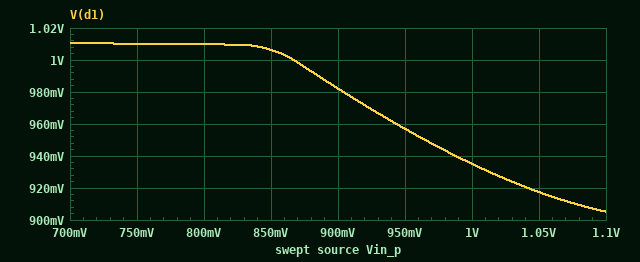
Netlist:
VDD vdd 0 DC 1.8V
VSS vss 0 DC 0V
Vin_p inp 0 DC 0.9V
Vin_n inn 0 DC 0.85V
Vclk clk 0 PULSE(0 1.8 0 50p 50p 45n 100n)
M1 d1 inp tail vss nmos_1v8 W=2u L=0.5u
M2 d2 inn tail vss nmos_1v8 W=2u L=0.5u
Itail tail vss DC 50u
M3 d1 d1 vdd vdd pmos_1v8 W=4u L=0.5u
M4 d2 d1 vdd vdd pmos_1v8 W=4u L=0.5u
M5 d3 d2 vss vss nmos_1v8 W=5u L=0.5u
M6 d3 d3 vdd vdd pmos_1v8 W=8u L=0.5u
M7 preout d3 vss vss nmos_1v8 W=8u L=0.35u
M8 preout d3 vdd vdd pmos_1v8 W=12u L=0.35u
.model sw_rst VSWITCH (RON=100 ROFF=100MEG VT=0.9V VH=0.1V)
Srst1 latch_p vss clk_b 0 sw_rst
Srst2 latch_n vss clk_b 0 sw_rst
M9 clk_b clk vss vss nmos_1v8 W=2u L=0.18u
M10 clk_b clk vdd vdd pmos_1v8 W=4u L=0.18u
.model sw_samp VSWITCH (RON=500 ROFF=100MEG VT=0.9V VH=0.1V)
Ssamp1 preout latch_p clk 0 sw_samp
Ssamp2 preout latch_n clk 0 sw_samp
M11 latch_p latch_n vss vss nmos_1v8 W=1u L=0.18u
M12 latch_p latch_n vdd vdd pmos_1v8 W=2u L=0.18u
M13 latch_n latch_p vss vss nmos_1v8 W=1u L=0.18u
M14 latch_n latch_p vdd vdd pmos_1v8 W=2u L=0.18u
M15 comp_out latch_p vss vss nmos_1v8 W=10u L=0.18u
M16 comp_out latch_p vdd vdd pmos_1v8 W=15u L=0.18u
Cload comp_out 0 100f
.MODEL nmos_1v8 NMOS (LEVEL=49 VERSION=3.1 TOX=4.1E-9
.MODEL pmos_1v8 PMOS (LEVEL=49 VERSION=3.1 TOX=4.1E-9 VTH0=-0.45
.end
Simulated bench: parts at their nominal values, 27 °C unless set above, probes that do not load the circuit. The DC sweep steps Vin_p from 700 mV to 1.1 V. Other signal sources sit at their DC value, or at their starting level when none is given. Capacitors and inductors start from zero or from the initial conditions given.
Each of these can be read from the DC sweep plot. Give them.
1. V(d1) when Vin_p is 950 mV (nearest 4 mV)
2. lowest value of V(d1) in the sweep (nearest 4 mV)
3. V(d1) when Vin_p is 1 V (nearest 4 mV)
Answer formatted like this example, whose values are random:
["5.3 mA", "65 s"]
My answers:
["956 mV", "904 mV", "936 mV"]
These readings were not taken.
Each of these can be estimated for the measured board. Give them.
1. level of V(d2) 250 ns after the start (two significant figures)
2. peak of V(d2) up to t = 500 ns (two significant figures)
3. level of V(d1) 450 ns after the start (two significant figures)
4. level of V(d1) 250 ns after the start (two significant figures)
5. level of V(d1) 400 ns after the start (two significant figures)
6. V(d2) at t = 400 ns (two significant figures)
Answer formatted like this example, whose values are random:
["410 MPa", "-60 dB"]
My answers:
["1.7 V", "1.7 V", "980 mV", "980 mV", "980 mV", "1.7 V"]
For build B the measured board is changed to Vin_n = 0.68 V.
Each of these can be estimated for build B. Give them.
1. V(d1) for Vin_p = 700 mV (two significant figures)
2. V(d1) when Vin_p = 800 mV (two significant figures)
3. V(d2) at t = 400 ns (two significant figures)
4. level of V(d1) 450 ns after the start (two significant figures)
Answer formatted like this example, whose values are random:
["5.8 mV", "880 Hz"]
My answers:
["1.0 V", "950 mV", "1.8 V", "910 mV"]
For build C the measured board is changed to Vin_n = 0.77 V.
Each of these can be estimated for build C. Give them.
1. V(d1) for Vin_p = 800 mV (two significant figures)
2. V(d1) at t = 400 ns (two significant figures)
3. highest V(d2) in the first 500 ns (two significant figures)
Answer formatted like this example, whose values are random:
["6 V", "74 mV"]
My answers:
["990 mV", "940 mV", "1.8 V"]
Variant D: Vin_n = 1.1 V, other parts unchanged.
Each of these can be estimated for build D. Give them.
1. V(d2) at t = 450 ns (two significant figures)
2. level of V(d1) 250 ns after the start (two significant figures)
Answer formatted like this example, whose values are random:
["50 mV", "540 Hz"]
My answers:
["290 mV", "1.0 V"]
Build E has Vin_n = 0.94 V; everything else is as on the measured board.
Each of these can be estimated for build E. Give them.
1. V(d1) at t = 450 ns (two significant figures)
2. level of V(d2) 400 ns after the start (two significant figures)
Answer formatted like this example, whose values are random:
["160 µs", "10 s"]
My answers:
["1.0 V", "360 mV"]
